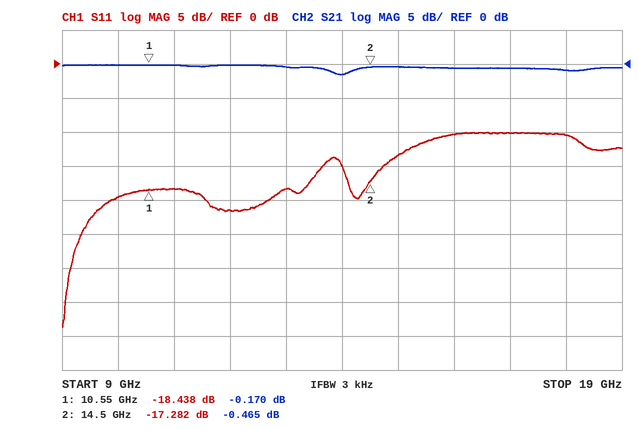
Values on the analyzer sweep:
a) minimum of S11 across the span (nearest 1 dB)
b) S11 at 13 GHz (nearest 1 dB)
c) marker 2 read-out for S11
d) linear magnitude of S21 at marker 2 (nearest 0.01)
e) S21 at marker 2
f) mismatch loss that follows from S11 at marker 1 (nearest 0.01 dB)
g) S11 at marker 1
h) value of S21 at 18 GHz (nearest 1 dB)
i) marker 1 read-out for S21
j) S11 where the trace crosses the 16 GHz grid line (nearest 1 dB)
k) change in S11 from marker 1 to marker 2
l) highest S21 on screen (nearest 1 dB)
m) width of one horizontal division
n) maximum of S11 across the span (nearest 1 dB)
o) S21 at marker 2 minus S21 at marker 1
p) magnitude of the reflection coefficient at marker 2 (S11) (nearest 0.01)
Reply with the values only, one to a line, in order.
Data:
-39 dB
-18 dB
-17.282 dB
0.95
-0.465 dB
0.06 dB
-18.438 dB
-1 dB
-0.170 dB
-10 dB
1.156 dB
0 dB
1 GHz
-10 dB
-0.295 dB
0.14
